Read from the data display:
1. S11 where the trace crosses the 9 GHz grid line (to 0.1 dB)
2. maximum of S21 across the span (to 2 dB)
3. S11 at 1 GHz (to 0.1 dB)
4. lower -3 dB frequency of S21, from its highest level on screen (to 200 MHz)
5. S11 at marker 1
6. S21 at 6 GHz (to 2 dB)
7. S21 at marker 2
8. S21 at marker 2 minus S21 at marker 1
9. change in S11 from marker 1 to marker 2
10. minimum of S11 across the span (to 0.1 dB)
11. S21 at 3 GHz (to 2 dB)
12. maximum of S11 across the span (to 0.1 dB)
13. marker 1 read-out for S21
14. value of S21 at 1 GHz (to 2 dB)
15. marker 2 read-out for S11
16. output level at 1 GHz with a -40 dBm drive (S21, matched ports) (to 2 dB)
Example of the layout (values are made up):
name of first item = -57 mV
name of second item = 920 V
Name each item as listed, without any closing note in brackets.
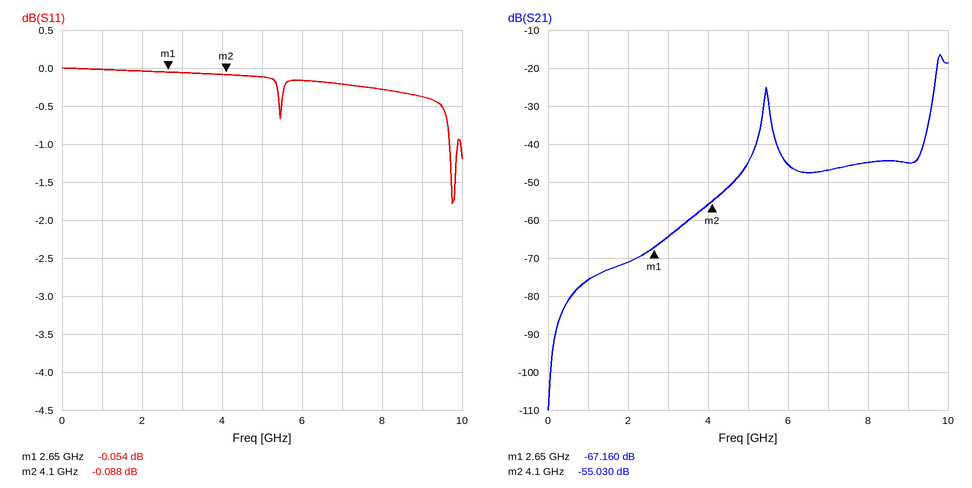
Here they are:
S11 where the trace crosses the 9 GHz grid line = -0.4 dB
maximum of S21 across the span = -16 dB
S11 at 1 GHz = 0.0 dB
lower -3 dB frequency of S21, from its highest level on screen = 9.8 GHz
S11 at marker 1 = -0.054 dB
S21 at 6 GHz = -46 dB
S21 at marker 2 = -55.030 dB
S21 at marker 2 minus S21 at marker 1 = 12.130 dB
change in S11 from marker 1 to marker 2 = -0.034 dB
minimum of S11 across the span = -1.8 dB
S21 at 3 GHz = -64 dB
maximum of S11 across the span = 0.0 dB
marker 1 read-out for S21 = -67.160 dB
value of S21 at 1 GHz = -76 dB
marker 2 read-out for S11 = -0.088 dB
output level at 1 GHz with a -40 dBm drive (S21, matched ports) = -116 dBm
